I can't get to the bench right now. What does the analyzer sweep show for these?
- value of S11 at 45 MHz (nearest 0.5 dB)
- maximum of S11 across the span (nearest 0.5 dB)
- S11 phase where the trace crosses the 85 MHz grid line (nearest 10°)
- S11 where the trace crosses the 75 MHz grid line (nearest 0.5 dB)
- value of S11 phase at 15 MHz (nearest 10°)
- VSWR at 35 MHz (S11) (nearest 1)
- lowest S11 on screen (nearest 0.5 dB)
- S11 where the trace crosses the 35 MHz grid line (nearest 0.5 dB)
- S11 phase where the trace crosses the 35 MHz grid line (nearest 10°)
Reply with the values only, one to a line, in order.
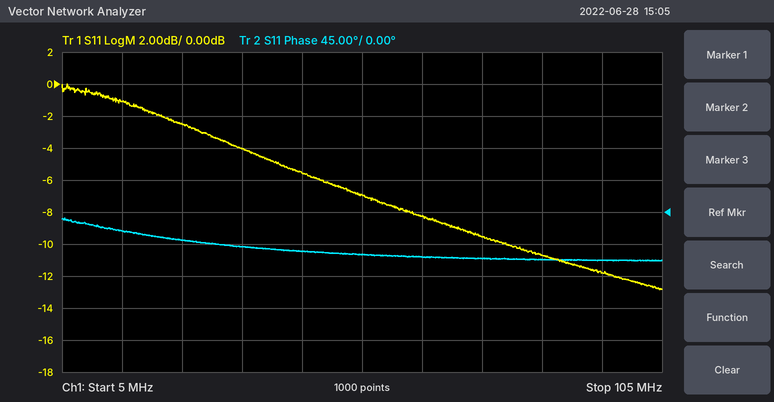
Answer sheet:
-5.5 dB
0.0 dB
-70°
-9.5 dB
-30°
4
-13.0 dB
-4.0 dB
-50°
